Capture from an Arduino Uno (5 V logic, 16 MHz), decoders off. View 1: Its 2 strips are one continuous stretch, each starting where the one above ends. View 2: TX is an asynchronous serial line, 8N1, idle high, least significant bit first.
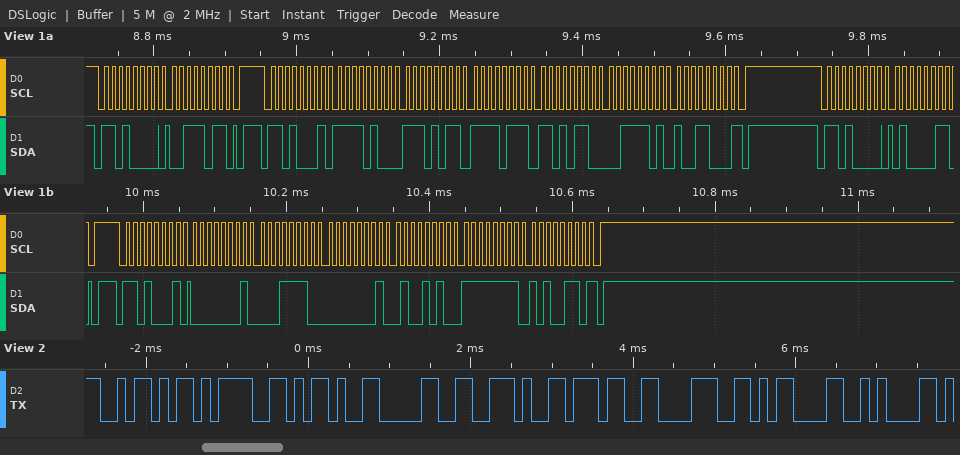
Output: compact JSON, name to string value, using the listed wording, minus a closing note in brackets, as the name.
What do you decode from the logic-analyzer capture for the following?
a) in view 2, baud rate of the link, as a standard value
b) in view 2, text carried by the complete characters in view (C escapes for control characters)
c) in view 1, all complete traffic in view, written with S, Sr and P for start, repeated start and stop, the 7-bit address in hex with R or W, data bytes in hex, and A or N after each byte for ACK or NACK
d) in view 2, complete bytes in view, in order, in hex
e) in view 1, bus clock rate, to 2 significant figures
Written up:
{"in view 2, baud rate of the link, as a standard value": "9600 baud", "in view 2, text carried by the complete characters in view": "\"Z=-0.78\\r\\n\"", "in view 1, all complete traffic in view, written with S, Sr and P for start, repeated start and stop, the 7-bit address in hex with R or W, data bytes in hex, and A or N after each byte for ACK or NACK": "S 68W A 3B A P S 68R A F4 A EB A F7 A D6 A 3D A 98 N P S 68W A 43 A P S 68R A 01 A 1E A 01 A 4A A FF A A6 N P", "in view 2, complete bytes in view, in order, in hex": "5A 3D 2D 30 2E 37 38 0D 0A", "in view 1, bus clock rate, to 2 significant figures": "100 kHz"}
